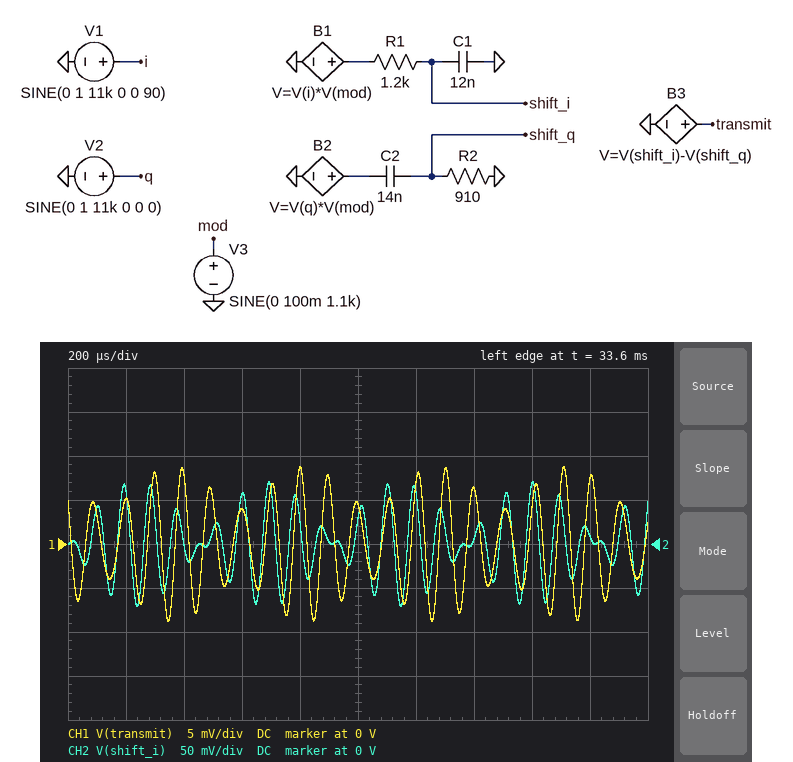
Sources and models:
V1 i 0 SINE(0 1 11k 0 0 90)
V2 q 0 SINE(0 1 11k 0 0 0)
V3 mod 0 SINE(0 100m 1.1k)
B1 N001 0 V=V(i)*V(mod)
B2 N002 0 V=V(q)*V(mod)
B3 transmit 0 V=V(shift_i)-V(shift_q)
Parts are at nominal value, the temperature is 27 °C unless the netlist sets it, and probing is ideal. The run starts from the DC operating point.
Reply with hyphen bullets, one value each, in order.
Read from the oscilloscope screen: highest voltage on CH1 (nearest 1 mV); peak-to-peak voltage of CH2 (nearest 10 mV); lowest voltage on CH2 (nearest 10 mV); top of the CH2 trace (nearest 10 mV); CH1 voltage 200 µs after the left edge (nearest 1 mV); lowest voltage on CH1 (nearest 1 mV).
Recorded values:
- 9 mV
- 140 mV
- -70 mV
- 70 mV
- 5 mV
- -9 mV
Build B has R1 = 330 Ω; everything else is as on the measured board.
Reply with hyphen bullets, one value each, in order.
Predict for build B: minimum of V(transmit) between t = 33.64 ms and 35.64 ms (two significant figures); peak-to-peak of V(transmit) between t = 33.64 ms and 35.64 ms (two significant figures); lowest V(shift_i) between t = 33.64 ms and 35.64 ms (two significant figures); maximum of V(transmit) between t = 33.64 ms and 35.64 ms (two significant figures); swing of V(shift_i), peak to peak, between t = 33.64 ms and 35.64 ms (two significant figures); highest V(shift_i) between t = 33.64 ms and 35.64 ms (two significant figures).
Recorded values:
- -47 mV
- 95 mV
- -96 mV
- 47 mV
- 190 mV
- 96 mV
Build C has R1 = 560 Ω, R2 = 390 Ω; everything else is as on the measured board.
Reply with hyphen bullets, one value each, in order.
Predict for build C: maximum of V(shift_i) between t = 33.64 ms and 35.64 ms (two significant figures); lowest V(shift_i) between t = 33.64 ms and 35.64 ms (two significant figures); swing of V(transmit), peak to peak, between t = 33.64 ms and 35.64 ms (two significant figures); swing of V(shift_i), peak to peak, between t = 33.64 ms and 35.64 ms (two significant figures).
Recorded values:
- 91 mV
- -91 mV
- 110 mV
- 180 mV
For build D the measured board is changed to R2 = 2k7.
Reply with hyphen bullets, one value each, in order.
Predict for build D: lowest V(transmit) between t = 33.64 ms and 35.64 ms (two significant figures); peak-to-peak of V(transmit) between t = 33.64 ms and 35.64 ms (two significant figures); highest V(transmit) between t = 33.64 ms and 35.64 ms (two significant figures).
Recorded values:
- -41 mV
- 82 mV
- 41 mV
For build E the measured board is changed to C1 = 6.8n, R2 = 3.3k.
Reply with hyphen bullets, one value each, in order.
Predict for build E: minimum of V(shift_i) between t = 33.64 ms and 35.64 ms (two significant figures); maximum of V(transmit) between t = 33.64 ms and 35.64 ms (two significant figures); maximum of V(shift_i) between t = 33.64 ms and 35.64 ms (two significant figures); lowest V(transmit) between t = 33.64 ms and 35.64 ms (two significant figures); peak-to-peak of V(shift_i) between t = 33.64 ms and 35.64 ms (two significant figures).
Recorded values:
- -87 mV
- 67 mV
- 87 mV
- -67 mV
- 170 mV
